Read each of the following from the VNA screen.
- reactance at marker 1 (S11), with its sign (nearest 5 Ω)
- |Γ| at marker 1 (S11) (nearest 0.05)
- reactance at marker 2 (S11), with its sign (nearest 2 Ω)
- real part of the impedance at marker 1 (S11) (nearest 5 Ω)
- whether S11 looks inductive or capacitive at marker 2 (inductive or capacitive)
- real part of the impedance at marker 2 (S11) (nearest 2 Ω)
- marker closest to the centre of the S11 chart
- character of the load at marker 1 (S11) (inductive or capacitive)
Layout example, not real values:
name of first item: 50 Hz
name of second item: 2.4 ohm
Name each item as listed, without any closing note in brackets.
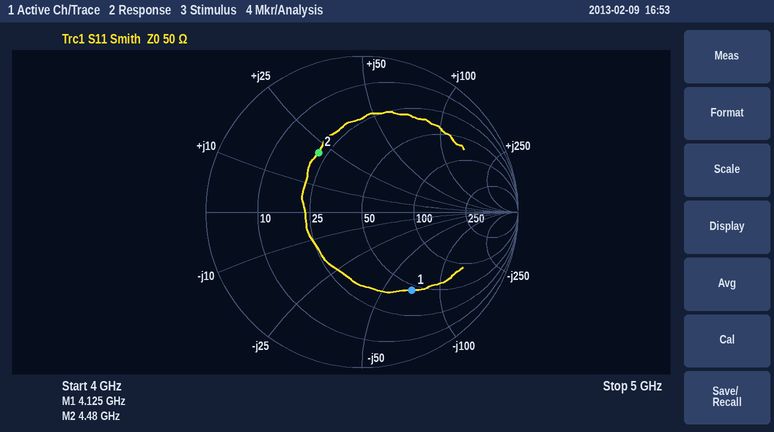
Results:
reactance at marker 1 (S11), with its sign: -70 Ω
|Γ| at marker 1 (S11): 0.60
reactance at marker 2 (S11), with its sign: +22 Ω
real part of the impedance at marker 1 (S11): 45 Ω
whether S11 looks inductive or capacitive at marker 2: inductive
real part of the impedance at marker 2 (S11): 22 Ω
marker closest to the centre of the S11 chart: marker 2
character of the load at marker 1 (S11): capacitive
